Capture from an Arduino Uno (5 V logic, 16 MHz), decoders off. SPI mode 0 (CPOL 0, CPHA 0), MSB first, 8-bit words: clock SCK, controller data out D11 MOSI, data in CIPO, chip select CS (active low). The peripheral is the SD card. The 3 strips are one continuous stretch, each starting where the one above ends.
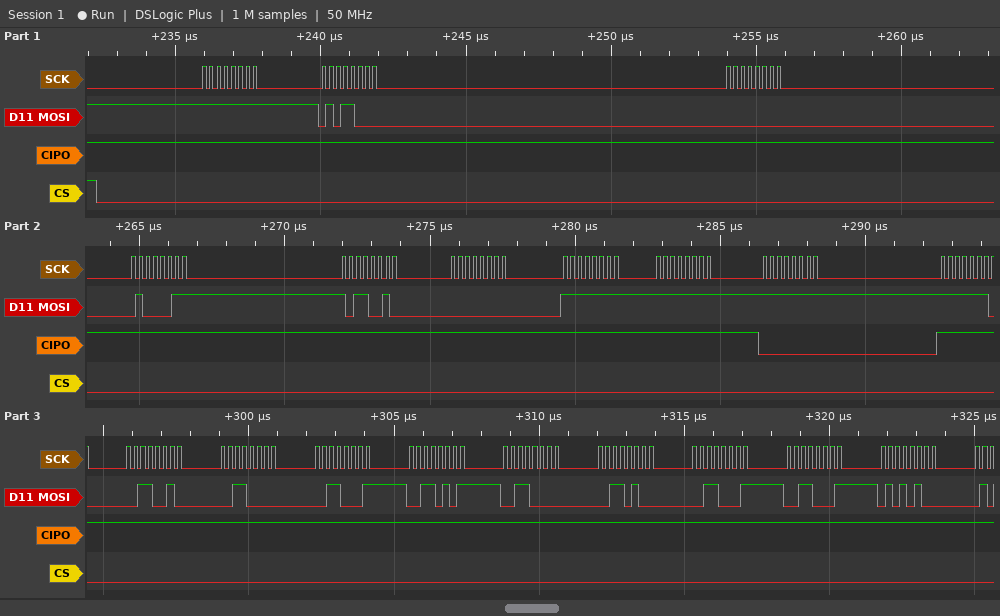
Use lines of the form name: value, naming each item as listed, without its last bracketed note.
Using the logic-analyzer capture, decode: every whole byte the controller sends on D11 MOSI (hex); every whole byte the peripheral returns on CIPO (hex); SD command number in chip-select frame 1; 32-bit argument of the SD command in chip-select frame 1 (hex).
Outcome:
every whole byte the controller sends on D11 MOSI: FF 58 00 43 B2 00 FF FF FF FE 32 30 31 35 30 34 31 31 54
every whole byte the peripheral returns on CIPO: FF FF FF FF FF FF FF FF 00 FF FF FF FF FF FF FF FF FF FF
SD command number in chip-select frame 1: CMD24
32-bit argument of the SD command in chip-select frame 1: 0x0043B200
